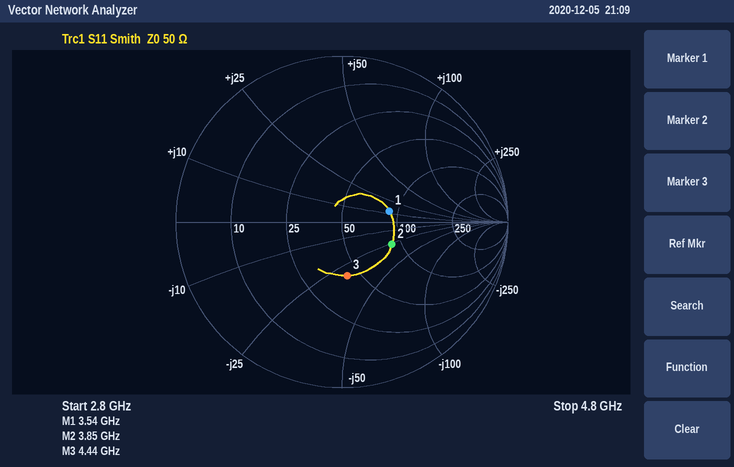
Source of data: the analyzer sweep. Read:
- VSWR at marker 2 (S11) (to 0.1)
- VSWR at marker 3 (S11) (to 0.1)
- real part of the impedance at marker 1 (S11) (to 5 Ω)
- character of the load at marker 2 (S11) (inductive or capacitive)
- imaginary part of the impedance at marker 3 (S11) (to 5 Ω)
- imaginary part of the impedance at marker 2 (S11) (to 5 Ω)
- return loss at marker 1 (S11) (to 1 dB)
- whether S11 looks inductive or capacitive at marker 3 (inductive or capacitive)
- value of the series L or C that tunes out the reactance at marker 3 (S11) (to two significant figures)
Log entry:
2.0
2.0
90 Ω
capacitive
-30 Ω
-25 Ω
11 dB
capacitive
1.1 nH
